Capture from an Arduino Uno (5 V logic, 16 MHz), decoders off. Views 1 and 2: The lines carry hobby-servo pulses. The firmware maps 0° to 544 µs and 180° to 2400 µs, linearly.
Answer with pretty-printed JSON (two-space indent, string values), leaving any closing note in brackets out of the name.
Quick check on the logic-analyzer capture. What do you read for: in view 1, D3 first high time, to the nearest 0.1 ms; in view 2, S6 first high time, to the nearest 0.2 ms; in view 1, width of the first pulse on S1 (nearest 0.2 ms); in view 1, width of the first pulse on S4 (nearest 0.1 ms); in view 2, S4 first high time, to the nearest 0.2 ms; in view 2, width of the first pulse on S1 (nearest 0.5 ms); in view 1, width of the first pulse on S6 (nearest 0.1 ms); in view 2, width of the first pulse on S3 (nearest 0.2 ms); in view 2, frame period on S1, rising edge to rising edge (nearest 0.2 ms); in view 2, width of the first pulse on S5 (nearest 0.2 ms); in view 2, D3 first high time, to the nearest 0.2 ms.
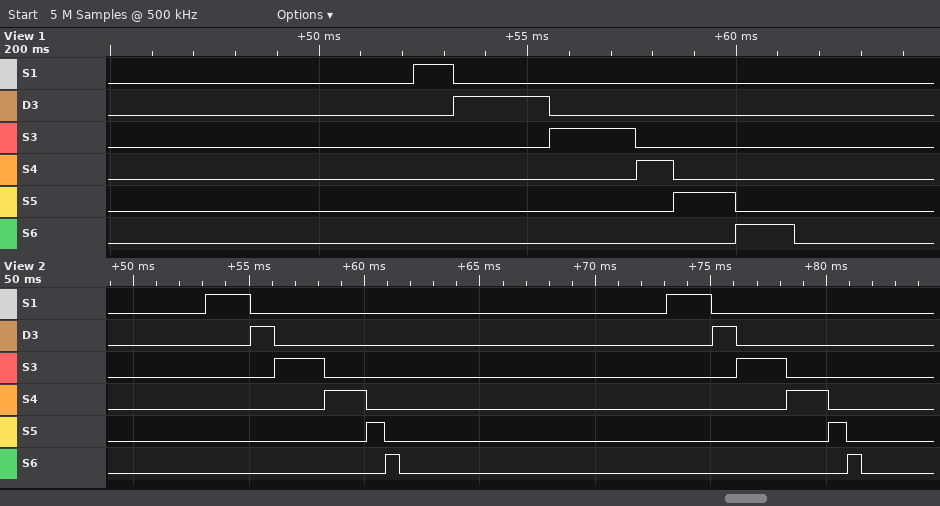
{
  "in view 1, D3 first high time, to the nearest 0.1 ms": "2.3 ms",
  "in view 2, S6 first high time, to the nearest 0.2 ms": "0.6 ms",
  "in view 1, width of the first pulse on S1": "1.0 ms",
  "in view 1, width of the first pulse on S4": "0.9 ms",
  "in view 2, S4 first high time, to the nearest 0.2 ms": "1.8 ms",
  "in view 2, width of the first pulse on S1": "2.0 ms",
  "in view 1, width of the first pulse on S6": "1.4 ms",
  "in view 2, width of the first pulse on S3": "2.2 ms",
  "in view 2, frame period on S1, rising edge to rising edge": "20.0 ms",
  "in view 2, width of the first pulse on S5": "0.8 ms",
  "in view 2, D3 first high time, to the nearest 0.2 ms": "1.0 ms"
}
